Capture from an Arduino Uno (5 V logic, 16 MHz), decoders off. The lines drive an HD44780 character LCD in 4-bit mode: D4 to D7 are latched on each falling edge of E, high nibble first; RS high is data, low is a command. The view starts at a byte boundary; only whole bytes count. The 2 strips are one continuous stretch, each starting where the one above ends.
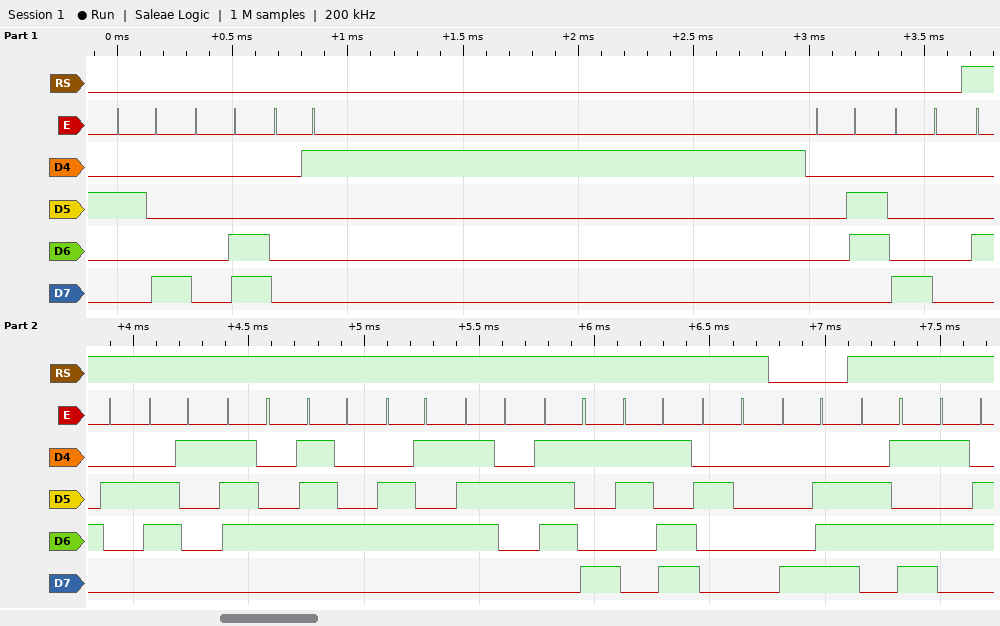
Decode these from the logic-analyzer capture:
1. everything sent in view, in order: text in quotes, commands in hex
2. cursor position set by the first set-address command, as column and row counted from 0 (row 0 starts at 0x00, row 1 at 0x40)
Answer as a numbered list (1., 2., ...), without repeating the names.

1. 0x28 0x0C 0x01 0x06 0x80 "Battery= " 0x8E "mV"
2. column 0, row 0
